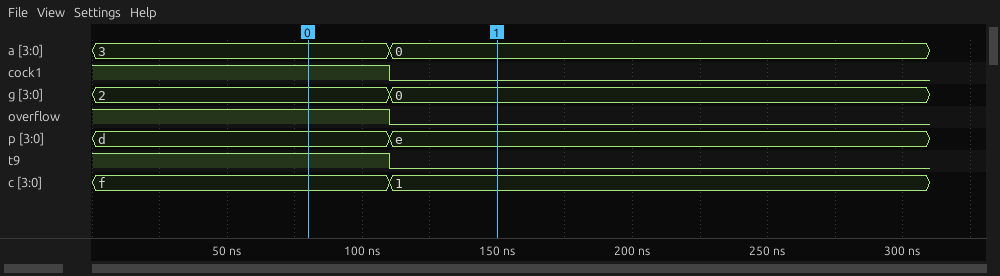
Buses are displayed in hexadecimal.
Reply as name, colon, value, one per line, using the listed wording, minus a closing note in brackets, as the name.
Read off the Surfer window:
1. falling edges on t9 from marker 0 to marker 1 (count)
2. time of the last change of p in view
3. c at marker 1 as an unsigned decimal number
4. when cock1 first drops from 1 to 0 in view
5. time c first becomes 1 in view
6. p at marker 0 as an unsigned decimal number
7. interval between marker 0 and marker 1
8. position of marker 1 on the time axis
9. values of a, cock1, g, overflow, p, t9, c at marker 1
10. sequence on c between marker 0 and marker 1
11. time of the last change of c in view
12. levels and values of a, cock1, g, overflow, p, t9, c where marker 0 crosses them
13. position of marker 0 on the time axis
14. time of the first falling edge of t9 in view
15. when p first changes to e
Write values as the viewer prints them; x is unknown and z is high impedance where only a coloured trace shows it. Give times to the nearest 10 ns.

falling edges on t9 from marker 0 to marker 1: 1
time of the last change of p in view: 110 ns
c at marker 1 as an unsigned decimal number: 1
when cock1 first drops from 1 to 0 in view: 110 ns
time c first becomes 1 in view: 110 ns
p at marker 0 as an unsigned decimal number: 13
interval between marker 0 and marker 1: 70 ns
position of marker 1 on the time axis: 150 ns
values of a, cock1, g, overflow, p, t9, c at marker 1: a=0, cock1=0, g=0, overflow=0, p=e, t9=0, c=1
sequence on c between marker 0 and marker 1: f, 1
time of the last change of c in view: 110 ns
levels and values of a, cock1, g, overflow, p, t9, c where marker 0 crosses them: a=3, cock1=1, g=2, overflow=1, p=d, t9=1, c=f
position of marker 0 on the time axis: 80 ns
time of the first falling edge of t9 in view: 110 ns
when p first changes to e: 110 ns
